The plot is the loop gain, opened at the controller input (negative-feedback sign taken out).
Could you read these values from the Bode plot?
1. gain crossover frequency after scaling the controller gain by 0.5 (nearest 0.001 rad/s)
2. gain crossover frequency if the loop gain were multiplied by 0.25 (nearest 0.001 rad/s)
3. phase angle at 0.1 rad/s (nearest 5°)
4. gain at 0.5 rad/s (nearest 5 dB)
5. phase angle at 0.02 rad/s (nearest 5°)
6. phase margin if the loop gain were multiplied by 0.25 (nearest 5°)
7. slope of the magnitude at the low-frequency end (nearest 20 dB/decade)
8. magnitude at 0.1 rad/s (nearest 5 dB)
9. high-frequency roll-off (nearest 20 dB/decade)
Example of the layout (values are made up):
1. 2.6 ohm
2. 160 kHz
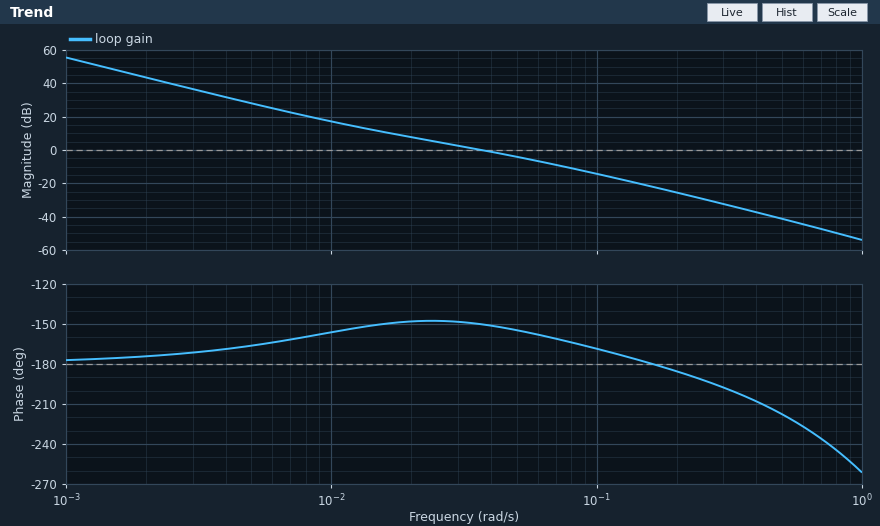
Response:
1. 0.023 rad/s
2. 0.014 rad/s
3. -170°
4. -40 dB
5. -150°
6. 30°
7. -40 dB/decade
8. -15 dB
9. -40 dB/decade
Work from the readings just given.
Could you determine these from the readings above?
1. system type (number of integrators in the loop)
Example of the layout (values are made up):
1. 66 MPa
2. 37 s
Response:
1. 2
